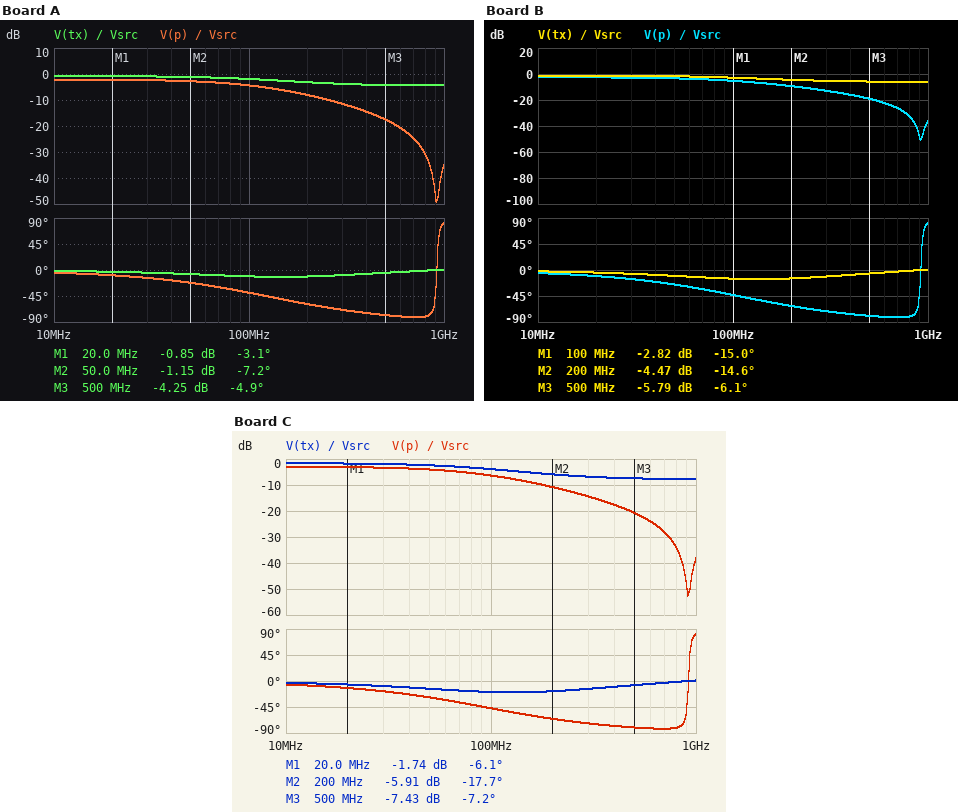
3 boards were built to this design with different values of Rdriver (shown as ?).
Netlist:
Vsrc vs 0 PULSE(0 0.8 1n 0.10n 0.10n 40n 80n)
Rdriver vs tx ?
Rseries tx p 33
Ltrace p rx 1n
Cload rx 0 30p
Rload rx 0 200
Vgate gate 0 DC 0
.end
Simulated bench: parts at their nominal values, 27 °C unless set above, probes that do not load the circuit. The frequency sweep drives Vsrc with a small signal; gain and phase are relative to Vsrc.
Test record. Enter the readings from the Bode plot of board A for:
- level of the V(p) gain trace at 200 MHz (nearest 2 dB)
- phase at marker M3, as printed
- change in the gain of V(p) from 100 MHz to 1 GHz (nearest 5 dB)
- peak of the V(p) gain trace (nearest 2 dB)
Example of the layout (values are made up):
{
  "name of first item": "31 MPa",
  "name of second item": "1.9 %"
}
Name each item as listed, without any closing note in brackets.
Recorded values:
{
  "level of the V(p) gain trace at 200 MHz": "-8 dB",
  "phase at marker M3, as printed": "-4.9 deg",
  "change in the gain of V(p) from 100 MHz to 1 GHz": "-30 dB",
  "peak of the V(p) gain trace": "-2 dB"
}
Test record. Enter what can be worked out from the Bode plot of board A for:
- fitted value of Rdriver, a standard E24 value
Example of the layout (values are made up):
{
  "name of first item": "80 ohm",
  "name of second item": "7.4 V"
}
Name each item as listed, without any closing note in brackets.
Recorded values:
{
  "fitted value of Rdriver, a standard E24 value": "22 Ω"
}
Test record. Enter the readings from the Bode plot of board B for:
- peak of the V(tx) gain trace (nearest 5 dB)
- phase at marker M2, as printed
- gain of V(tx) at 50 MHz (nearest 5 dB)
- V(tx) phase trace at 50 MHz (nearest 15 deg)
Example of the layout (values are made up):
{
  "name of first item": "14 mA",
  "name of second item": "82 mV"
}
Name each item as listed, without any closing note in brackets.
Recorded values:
{
  "peak of the V(tx) gain trace": "0 dB",
  "phase at marker M2, as printed": "-14.6 deg",
  "gain of V(tx) at 50 MHz": "0 dB",
  "V(tx) phase trace at 50 MHz": "-15 deg"
}
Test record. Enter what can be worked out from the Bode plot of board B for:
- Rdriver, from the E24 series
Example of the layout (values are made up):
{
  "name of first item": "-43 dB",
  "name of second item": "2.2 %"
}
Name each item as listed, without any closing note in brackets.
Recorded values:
{
  "Rdriver, from the E24 series": "33 Ω"
}
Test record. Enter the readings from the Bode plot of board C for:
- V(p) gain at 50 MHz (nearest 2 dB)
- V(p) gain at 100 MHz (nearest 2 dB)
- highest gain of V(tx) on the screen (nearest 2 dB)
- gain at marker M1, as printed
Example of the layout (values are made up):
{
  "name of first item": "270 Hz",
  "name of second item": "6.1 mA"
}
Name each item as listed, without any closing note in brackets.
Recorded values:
{
  "V(p) gain at 50 MHz": "-4 dB",
  "V(p) gain at 100 MHz": "-6 dB",
  "highest gain of V(tx) on the screen": "-2 dB",
  "gain at marker M1, as printed": "-1.74 dB"
}
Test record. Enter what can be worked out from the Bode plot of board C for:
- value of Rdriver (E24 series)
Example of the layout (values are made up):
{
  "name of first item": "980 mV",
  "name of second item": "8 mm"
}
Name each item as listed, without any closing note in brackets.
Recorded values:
{
  "value of Rdriver": "47 Ω"
}
